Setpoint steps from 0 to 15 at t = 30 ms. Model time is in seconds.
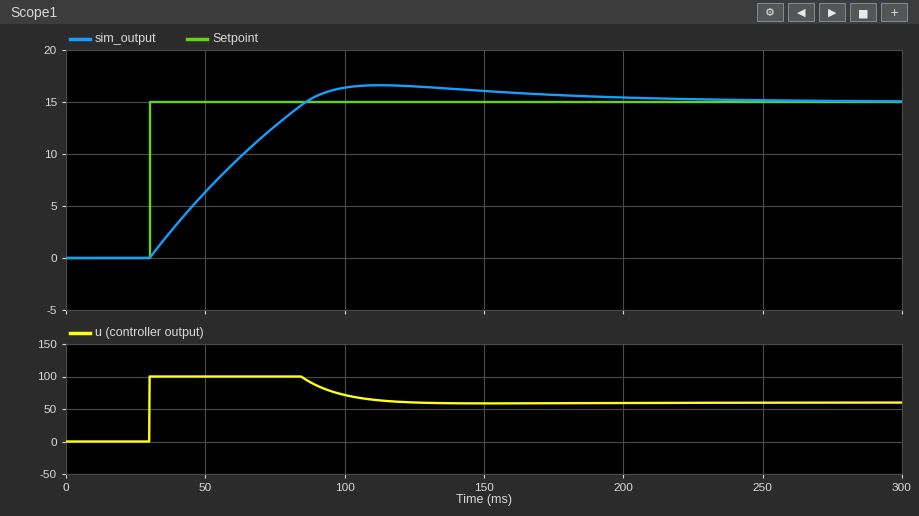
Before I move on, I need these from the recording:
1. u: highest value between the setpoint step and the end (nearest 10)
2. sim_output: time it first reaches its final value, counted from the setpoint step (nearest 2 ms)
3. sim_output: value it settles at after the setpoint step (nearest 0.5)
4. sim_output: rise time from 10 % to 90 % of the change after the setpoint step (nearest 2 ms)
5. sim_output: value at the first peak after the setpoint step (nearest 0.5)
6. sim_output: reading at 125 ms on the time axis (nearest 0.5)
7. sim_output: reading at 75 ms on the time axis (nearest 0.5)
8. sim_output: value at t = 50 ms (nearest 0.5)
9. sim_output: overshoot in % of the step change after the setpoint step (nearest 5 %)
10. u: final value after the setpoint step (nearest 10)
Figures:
100
56 ms
15.0
44 ms
16.5
16.5
12.5
6.5
10 %
60
